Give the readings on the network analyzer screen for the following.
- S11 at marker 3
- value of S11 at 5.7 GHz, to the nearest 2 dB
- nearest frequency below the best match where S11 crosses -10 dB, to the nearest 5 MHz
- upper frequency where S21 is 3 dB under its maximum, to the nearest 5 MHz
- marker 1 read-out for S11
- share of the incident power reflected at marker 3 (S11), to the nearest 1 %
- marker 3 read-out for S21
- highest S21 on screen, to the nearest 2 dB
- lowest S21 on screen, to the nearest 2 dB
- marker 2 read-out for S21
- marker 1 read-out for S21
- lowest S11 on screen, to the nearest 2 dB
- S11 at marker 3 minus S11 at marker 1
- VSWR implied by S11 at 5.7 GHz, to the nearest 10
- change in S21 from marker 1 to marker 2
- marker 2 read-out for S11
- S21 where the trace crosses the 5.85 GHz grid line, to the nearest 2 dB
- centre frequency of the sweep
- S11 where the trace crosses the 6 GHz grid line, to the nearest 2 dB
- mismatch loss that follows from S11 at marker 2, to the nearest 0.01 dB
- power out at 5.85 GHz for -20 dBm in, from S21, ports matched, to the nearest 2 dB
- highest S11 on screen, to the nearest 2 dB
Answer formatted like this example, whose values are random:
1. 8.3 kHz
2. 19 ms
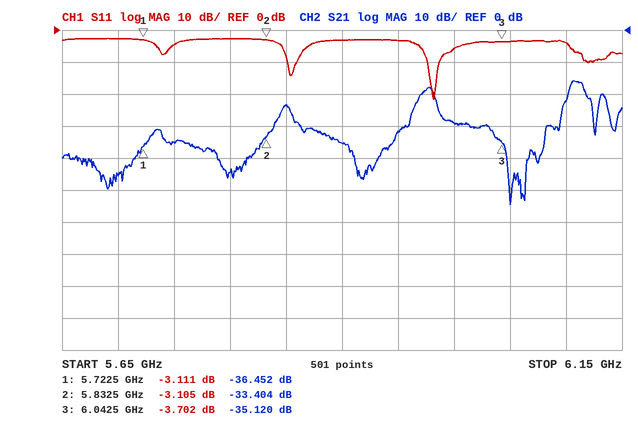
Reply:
1. -3.702 dB
2. -2 dB
3. 5.975 GHz
4. 6.115 GHz
5. -3.111 dB
6. 43 %
7. -35.120 dB
8. -16 dB
9. -54 dB
10. -33.404 dB
11. -36.452 dB
12. -22 dB
13. -0.591 dB
14. 10
15. 3.048 dB
16. -3.105 dB
17. -24 dB
18. 5.9 GHz
19. -6 dB
20. 2.92 dB
21. -44 dBm
22. -2 dB
